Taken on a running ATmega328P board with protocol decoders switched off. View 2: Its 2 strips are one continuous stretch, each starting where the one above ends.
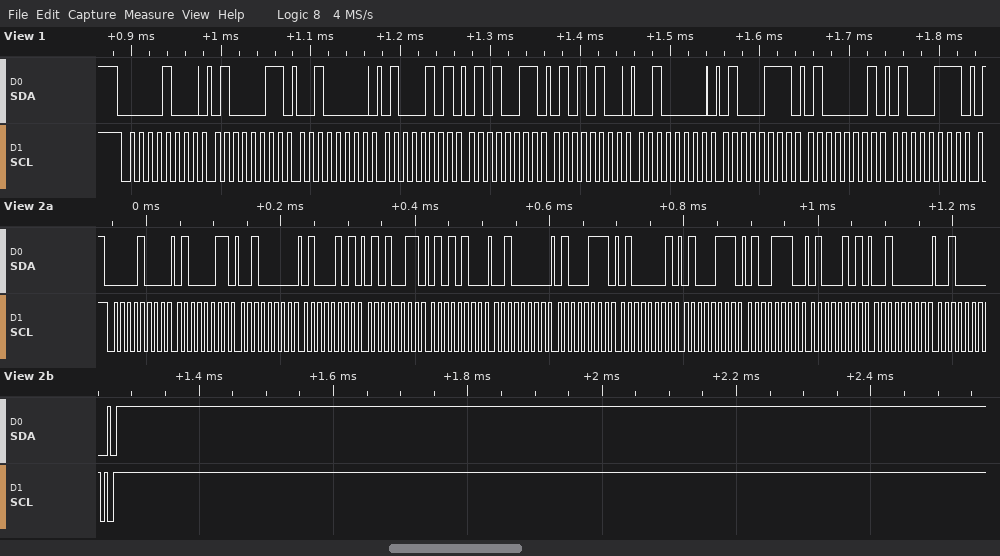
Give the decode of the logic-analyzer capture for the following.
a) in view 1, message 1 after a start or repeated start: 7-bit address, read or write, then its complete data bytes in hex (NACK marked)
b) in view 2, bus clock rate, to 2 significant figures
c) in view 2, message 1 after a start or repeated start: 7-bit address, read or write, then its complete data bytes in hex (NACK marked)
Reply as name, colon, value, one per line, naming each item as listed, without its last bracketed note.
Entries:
in view 1, message 1 after a start or repeated start: 7-bit address, read or write, then its complete data bytes in hex: 0x04 write: 43 20 45 53 54 20 47 41 47
in view 2, bus clock rate, to 2 significant figures: 100 kHz
in view 2, message 1 after a start or repeated start: 7-bit address, read or write, then its complete data bytes in hex: 0x04 write: 43 20 45 53 54 20 47 41 47 4E 45 20 20
